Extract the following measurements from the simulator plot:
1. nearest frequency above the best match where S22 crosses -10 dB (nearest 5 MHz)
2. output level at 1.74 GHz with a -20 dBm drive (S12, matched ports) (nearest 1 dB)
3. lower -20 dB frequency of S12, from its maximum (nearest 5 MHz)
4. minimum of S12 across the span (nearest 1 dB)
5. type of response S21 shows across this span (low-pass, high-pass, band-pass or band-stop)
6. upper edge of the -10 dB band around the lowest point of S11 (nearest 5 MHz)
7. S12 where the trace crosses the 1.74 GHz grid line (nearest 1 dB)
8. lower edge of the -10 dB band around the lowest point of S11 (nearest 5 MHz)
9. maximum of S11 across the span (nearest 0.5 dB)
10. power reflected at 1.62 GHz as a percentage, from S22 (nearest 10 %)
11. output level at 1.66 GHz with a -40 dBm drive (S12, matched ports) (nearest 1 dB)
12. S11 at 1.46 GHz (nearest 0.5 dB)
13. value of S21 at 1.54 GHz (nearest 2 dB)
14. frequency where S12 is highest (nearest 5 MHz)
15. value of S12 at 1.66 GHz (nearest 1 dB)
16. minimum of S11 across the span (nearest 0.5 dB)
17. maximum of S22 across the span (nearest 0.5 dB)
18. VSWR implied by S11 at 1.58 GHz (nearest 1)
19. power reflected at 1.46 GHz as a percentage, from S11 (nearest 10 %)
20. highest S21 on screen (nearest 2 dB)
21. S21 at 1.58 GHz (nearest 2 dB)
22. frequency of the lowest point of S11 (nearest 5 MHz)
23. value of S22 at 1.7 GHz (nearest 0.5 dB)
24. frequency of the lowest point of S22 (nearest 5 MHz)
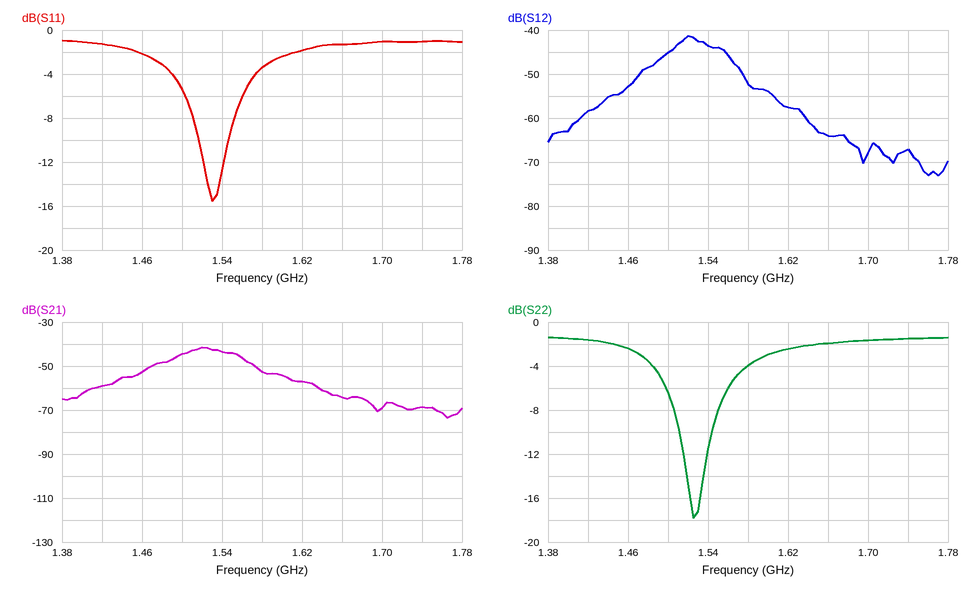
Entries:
1.545 GHz
-87 dBm
1.405 GHz
-73 dB
band-pass
1.545 GHz
-67 dB
1.515 GHz
-1.0 dB
60 %
-104 dBm
-2.0 dB
-44 dB
1.520 GHz
-64 dB
-15.5 dB
-1.5 dB
5
60 %
-42 dB
-52 dB
1.530 GHz
-1.5 dB
1.525 GHz
